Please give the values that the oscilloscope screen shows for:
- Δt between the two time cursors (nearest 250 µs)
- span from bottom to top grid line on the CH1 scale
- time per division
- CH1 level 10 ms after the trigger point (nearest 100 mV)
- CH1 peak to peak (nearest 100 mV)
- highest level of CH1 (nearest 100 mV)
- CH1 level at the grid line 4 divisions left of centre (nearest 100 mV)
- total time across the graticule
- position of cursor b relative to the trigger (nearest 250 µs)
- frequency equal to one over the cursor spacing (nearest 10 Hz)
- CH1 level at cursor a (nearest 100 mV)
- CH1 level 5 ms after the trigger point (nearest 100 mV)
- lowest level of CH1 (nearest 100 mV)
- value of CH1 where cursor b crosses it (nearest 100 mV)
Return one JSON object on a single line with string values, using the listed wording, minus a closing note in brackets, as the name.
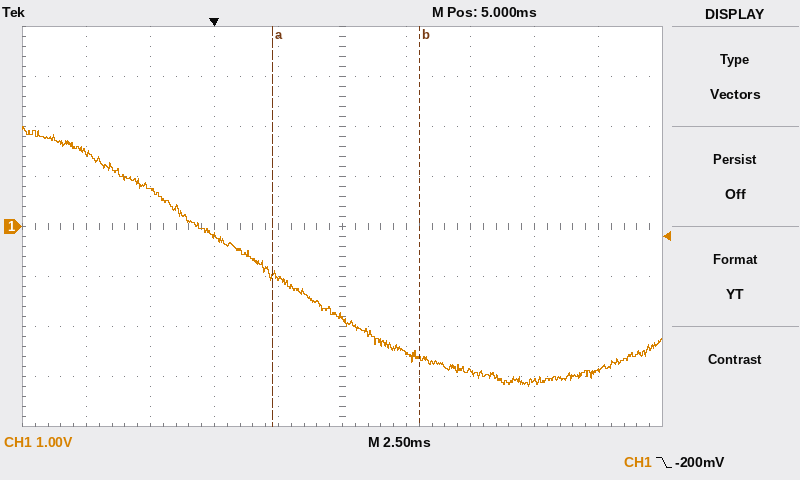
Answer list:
{"Δt between the two time cursors": "5.75 ms", "span from bottom to top grid line on the CH1 scale": "8 V", "time per division": "2.5 ms", "CH1 level 10 ms after the trigger point": "-2.9 V", "CH1 peak to peak": "5.2 V", "highest level of CH1": "2.0 V", "CH1 level at the grid line 4 divisions left of centre": "1.5 V", "total time across the graticule": "25 ms", "position of cursor b relative to the trigger": "+8.00 ms", "frequency equal to one over the cursor spacing": "170 Hz", "CH1 level at cursor a": "-1.0 V", "CH1 level 5 ms after the trigger point": "-1.8 V", "lowest level of CH1": "-3.2 V", "value of CH1 where cursor b crosses it": "-2.6 V"}
